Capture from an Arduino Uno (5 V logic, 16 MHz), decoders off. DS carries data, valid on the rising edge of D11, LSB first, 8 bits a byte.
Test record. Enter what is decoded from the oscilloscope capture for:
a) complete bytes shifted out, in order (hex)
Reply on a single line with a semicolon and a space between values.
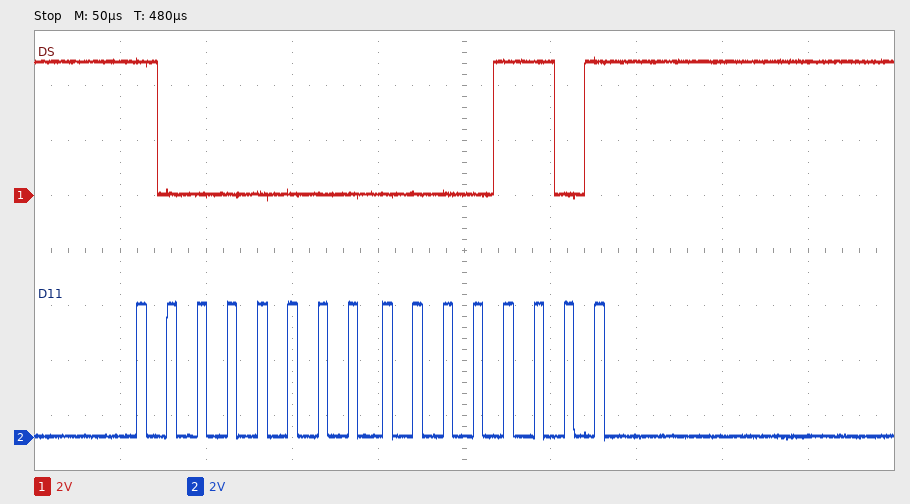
0x01 0xB0
